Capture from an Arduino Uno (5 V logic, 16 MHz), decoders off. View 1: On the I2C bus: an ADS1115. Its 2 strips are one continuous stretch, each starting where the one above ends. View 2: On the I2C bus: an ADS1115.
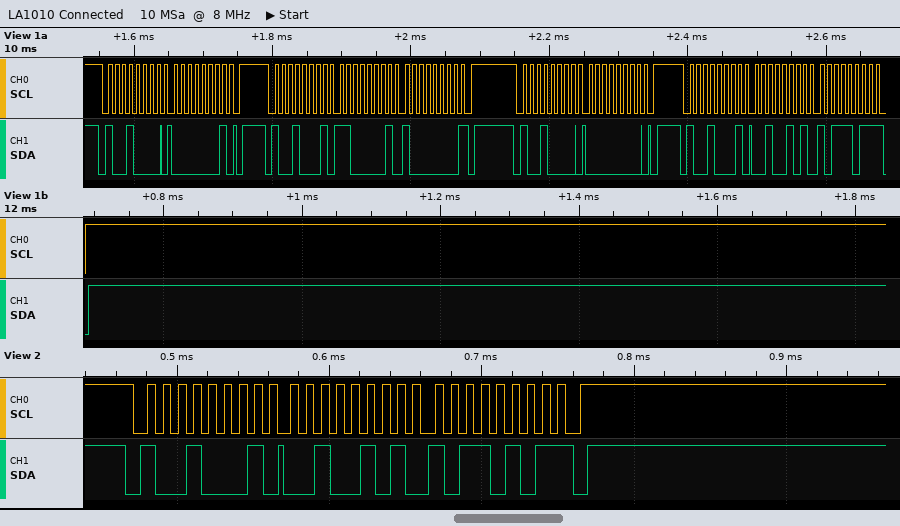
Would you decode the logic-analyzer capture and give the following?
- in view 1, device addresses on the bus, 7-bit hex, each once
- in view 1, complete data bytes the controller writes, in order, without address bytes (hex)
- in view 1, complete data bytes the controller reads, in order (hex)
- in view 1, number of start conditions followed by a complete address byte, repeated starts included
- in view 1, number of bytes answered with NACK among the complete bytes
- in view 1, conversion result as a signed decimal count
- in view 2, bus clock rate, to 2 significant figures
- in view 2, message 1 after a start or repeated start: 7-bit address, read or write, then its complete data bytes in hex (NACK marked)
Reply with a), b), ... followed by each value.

a) 0x48
b) 01 00
c) C1 80 25 BB
d) 4
e) 2
f) 9659
g) 100 kHz
h) 0x48 read: 25 B5 NACK
